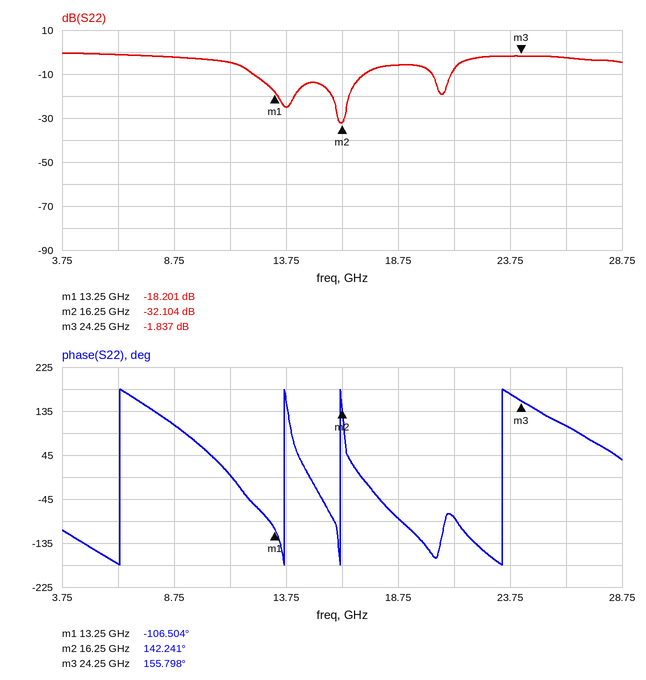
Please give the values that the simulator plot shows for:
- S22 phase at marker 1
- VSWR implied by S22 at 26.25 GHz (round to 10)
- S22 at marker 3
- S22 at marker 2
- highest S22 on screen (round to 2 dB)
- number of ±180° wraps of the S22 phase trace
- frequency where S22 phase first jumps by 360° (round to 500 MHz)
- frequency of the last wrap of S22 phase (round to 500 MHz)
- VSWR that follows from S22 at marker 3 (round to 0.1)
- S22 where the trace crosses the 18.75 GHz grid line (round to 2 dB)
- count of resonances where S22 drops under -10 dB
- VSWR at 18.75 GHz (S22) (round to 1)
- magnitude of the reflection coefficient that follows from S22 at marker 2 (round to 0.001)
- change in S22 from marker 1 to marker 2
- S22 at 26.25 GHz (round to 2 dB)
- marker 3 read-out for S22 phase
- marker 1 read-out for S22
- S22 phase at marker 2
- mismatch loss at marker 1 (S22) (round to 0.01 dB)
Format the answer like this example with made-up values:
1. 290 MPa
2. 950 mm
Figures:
1. -106.504°
2. 10
3. -1.837 dB
4. -32.104 dB
5. 0 dB
6. 4
7. 6.5 GHz
8. 23.5 GHz
9. 9.5
10. -6 dB
11. 3
12. 3
13. 0.025
14. -13.903 dB
15. -2 dB
16. 155.798°
17. -18.201 dB
18. 142.241°
19. 0.07 dB
